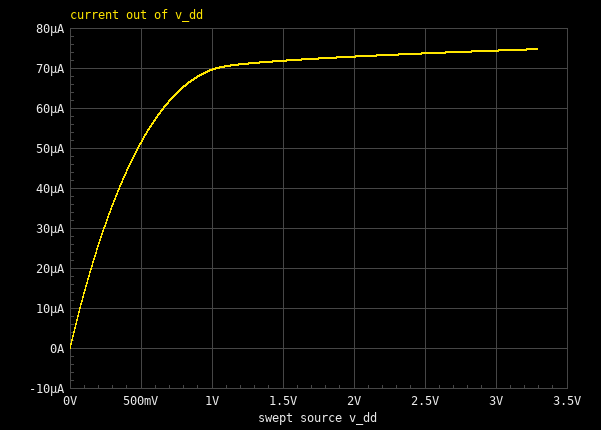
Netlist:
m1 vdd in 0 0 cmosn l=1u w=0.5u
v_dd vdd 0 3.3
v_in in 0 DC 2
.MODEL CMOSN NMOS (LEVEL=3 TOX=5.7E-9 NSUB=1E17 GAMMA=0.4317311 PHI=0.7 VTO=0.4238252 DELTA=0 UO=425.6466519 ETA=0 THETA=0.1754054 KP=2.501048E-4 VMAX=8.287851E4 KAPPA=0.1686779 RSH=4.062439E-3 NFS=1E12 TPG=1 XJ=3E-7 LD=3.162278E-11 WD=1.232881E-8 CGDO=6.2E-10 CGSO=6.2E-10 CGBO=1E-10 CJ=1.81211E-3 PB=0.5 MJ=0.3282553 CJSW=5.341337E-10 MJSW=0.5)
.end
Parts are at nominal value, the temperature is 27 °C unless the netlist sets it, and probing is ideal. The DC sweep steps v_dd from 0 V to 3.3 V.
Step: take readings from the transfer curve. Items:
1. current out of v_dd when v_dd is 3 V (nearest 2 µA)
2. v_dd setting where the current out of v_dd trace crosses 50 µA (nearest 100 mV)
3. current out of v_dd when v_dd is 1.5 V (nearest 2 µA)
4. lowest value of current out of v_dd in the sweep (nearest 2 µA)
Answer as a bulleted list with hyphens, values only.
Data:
- 74 µA
- 500 mV
- 72 µA
- 0 A
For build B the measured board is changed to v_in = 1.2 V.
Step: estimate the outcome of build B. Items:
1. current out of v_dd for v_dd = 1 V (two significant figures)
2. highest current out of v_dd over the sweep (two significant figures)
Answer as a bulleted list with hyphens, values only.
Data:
- 24 µA
- 25 µA
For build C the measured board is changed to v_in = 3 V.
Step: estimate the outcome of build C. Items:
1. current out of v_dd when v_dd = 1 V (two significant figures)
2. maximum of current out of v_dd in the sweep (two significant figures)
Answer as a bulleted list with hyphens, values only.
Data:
- 120 µA
- 150 µA
